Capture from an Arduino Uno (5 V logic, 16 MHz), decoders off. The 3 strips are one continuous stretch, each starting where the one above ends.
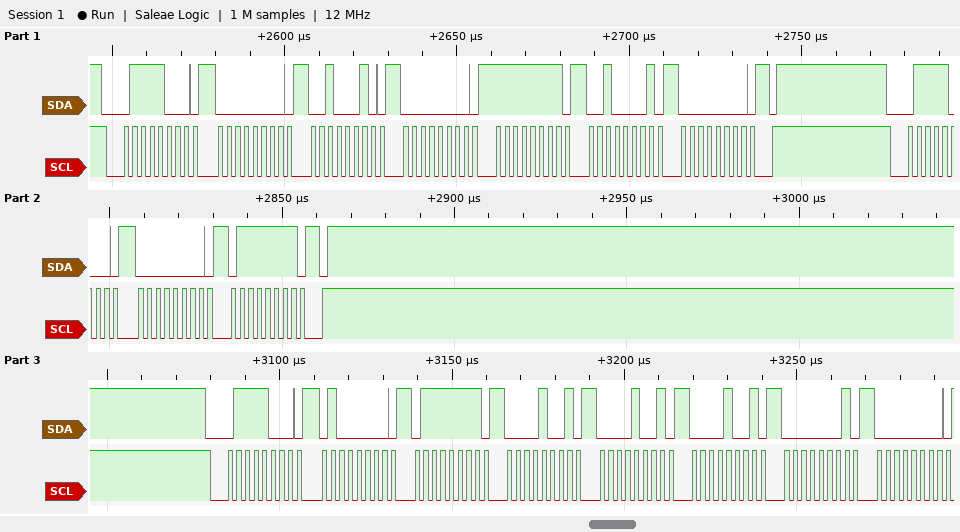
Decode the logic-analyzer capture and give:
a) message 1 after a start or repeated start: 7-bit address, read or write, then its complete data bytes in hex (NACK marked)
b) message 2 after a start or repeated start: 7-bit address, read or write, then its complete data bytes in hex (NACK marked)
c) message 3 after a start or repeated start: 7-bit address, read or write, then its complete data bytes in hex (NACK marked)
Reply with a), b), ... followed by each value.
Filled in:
a) 0x3C write: 00 22 00 FF 21 00
b) 0x3C write: 00 7F
c) 0x3C write: 40 7F 09 09 09 01 00
